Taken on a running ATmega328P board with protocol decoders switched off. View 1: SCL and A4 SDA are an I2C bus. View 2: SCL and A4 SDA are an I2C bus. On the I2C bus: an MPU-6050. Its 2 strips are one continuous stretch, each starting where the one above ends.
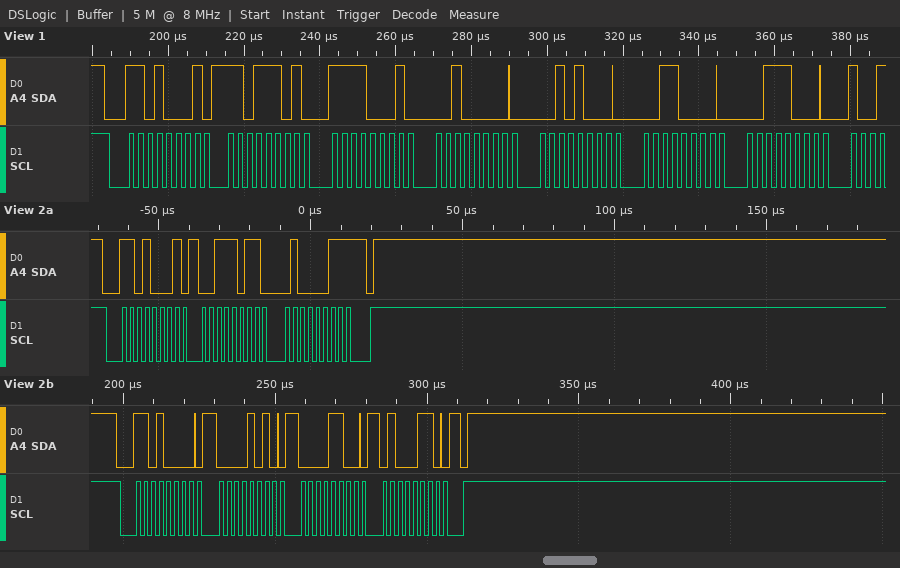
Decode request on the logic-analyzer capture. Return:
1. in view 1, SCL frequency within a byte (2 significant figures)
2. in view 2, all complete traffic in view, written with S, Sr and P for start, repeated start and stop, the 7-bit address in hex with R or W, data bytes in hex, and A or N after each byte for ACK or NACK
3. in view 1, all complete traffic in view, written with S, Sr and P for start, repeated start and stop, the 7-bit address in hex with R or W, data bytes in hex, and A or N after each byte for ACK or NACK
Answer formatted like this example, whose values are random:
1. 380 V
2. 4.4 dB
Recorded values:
1. 400 kHz
2. S 68R A 3B A 43 N P S 68W A 0A A 0C A 46 A P
3. S 68R A DD A F1 A 20 A 28 A 30 A 38 A
